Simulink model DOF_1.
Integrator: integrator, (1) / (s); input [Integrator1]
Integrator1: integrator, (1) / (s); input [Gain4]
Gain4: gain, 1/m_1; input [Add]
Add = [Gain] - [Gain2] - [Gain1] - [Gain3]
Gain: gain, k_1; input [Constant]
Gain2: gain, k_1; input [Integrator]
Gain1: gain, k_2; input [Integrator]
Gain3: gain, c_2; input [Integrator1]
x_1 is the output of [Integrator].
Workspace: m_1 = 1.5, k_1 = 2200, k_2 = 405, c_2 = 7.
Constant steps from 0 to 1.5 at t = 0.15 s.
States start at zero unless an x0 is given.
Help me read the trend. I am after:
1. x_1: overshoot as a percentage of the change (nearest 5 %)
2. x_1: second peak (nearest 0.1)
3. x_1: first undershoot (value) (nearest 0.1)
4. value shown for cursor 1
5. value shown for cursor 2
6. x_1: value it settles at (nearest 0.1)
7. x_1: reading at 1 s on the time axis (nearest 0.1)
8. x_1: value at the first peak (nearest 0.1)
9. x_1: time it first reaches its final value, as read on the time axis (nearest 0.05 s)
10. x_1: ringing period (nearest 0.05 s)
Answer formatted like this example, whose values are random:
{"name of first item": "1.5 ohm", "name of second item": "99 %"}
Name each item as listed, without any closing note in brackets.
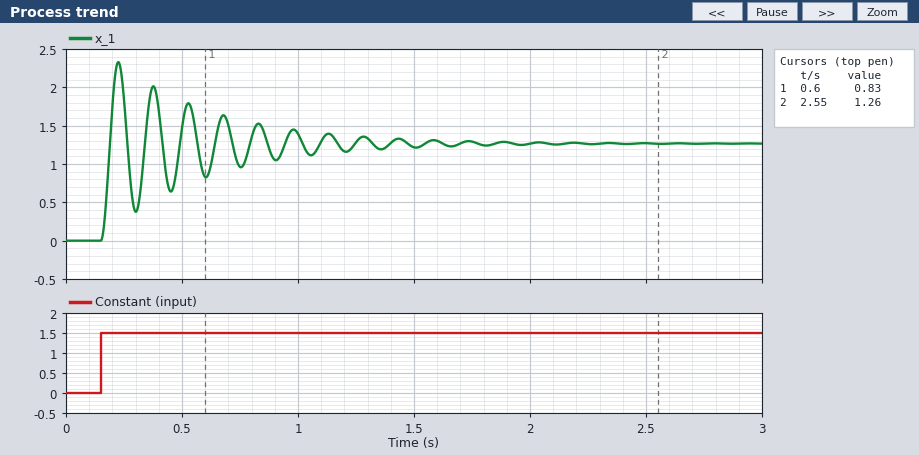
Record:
{"x_1: overshoot as a percentage of the change": "85 %", "x_1: second peak": "2.0", "x_1: first undershoot (value)": "0.4", "value shown for cursor 1": "0.83", "value shown for cursor 2": "1.26", "x_1: value it settles at": "1.3", "x_1: reading at 1 s on the time axis": "1.4", "x_1: value at the first peak": "2.3", "x_1: time it first reaches its final value, as read on the time axis": "0.20 s", "x_1: ringing period": "0.15 s"}
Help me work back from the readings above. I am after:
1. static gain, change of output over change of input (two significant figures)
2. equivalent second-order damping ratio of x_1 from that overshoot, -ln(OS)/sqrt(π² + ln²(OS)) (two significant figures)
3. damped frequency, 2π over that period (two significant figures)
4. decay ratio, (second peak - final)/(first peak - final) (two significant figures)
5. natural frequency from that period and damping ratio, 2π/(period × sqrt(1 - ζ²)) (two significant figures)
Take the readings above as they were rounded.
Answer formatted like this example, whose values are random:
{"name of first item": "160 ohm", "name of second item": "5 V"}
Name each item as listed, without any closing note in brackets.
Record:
{"static gain, change of output over change of input": "0.87", "equivalent second-order damping ratio of x_1 from that overshoot, -ln(OS)/sqrt(π² + ln²(OS))": "0.052", "damped frequency, 2π over that period": "42 rad/s", "decay ratio, (second peak - final)/(first peak - final)": "0.70", "natural frequency from that period and damping ratio, 2π/(period × sqrt(1 - ζ²))": "42 rad/s"}
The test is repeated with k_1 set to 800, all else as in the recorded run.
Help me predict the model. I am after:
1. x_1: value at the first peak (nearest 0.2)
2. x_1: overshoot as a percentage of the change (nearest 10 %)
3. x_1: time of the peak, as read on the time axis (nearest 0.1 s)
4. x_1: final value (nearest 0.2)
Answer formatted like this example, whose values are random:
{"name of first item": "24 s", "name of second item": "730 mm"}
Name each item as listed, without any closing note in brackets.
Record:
{"x_1: value at the first peak": "1.8", "x_1: overshoot as a percentage of the change": "80 %", "x_1: time of the peak, as read on the time axis": "0.3 s", "x_1: final value": "1.0"}
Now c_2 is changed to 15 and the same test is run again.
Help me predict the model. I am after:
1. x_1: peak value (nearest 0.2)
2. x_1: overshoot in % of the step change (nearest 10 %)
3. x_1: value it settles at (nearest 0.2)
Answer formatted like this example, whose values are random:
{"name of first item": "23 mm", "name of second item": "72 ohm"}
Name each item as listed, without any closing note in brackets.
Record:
{"x_1: peak value": "2.2", "x_1: overshoot in % of the step change": "70 %", "x_1: value it settles at": "1.2"}
